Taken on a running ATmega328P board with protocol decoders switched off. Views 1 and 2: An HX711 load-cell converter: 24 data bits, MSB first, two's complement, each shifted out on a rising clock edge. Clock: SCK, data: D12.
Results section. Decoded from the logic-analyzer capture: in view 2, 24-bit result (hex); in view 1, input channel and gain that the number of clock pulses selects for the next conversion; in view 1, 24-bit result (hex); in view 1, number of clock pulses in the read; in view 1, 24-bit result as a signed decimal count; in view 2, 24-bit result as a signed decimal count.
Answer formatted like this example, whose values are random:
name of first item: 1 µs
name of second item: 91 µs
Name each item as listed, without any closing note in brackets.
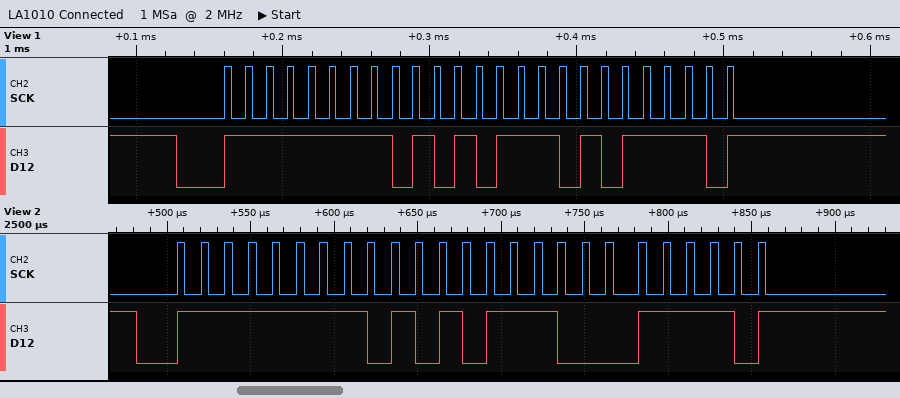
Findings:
in view 2, 24-bit result: 0xFF571E
in view 1, input channel and gain that the number of clock pulses selects for the next conversion: channel A, gain 128
in view 1, 24-bit result: 0xFF575E
in view 1, number of clock pulses in the read: 25
in view 1, 24-bit result as a signed decimal count: -43170
in view 2, 24-bit result as a signed decimal count: -43234
